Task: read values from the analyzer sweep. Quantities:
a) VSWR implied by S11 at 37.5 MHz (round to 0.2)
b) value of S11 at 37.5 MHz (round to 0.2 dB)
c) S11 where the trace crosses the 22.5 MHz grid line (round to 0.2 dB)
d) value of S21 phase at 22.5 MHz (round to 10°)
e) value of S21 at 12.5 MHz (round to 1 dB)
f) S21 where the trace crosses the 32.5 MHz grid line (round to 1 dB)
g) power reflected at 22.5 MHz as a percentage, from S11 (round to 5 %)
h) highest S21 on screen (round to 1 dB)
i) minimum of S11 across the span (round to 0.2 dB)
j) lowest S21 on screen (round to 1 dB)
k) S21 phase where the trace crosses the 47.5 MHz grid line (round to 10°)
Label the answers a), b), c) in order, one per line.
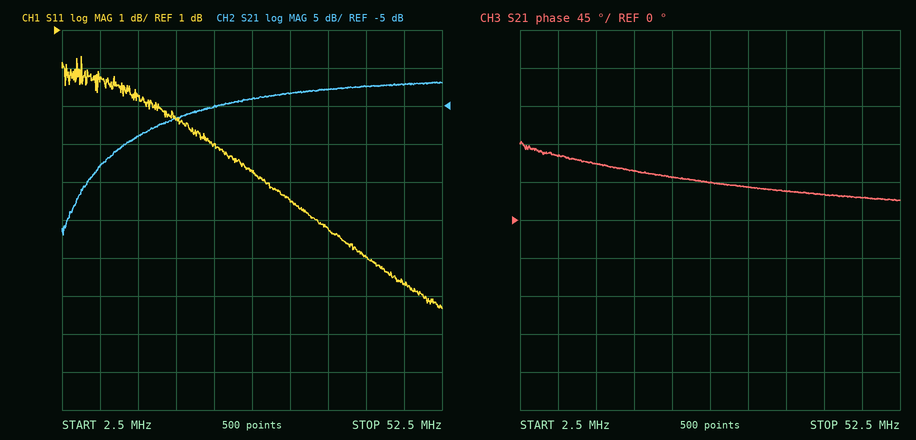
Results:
a) 4.2
b) -4.2 dB
c) -2.0 dB
d) 50°
e) -9 dB
f) -3 dB
g) 65 %
h) -2 dB
i) -6.4 dB
j) -22 dB
k) 30°
